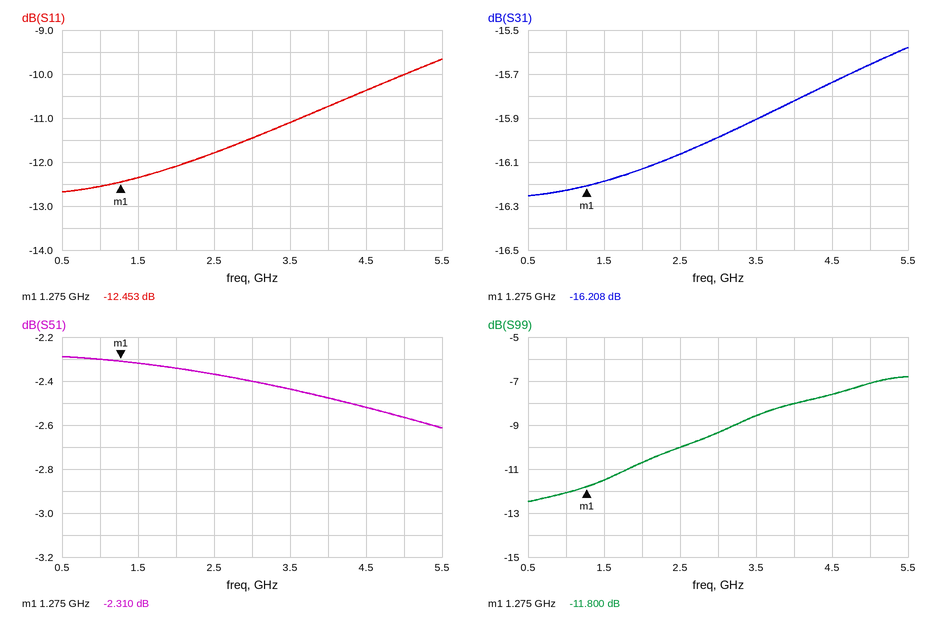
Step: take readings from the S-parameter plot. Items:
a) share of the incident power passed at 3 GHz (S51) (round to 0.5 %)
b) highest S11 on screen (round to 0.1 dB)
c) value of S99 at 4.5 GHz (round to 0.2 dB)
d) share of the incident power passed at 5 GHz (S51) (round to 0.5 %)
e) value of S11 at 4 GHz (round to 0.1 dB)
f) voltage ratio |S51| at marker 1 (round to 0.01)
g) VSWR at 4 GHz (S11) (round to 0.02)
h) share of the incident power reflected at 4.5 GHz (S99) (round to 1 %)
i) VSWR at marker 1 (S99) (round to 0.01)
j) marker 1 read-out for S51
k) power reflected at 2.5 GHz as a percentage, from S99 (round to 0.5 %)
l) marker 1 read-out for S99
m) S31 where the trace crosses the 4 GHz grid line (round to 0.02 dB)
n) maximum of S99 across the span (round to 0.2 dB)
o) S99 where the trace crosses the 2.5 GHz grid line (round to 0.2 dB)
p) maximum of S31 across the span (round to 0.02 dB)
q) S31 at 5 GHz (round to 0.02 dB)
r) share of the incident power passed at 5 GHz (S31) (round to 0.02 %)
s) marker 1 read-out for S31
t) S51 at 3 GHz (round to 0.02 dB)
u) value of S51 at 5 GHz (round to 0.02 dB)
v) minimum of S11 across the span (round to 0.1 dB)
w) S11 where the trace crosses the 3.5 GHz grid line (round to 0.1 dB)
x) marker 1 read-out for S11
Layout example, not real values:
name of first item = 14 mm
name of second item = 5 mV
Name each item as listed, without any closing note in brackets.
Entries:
share of the incident power passed at 3 GHz (S51) = 57.5 %
highest S11 on screen = -9.7 dB
value of S99 at 4.5 GHz = -7.6 dB
share of the incident power passed at 5 GHz (S51) = 55.5 %
value of S11 at 4 GHz = -10.7 dB
voltage ratio |S51| at marker 1 = 0.77
VSWR at 4 GHz (S11) = 1.82
share of the incident power reflected at 4.5 GHz (S99) = 17 %
VSWR at marker 1 (S99) = 1.69
marker 1 read-out for S51 = -2.310 dB
power reflected at 2.5 GHz as a percentage, from S99 = 10.0 %
marker 1 read-out for S99 = -11.800 dB
S31 where the trace crosses the 4 GHz grid line = -15.82 dB
maximum of S99 across the span = -6.8 dB
S99 where the trace crosses the 2.5 GHz grid line = -10.0 dB
maximum of S31 across the span = -15.58 dB
S31 at 5 GHz = -15.66 dB
share of the incident power passed at 5 GHz (S31) = 2.72 %
marker 1 read-out for S31 = -16.208 dB
S51 at 3 GHz = -2.40 dB
value of S51 at 5 GHz = -2.56 dB
minimum of S11 across the span = -12.7 dB
S11 where the trace crosses the 3.5 GHz grid line = -11.1 dB
marker 1 read-out for S11 = -12.453 dB
